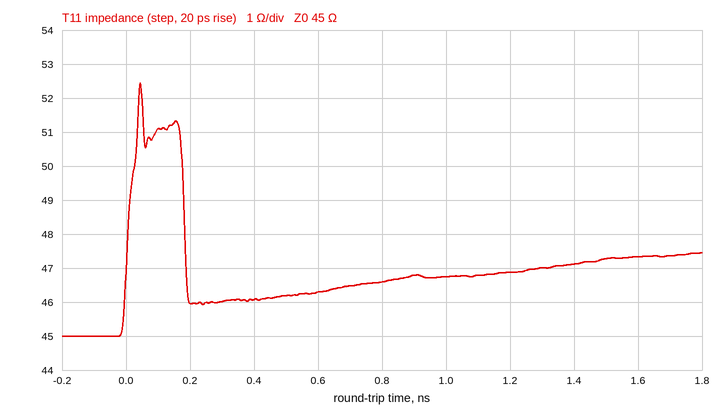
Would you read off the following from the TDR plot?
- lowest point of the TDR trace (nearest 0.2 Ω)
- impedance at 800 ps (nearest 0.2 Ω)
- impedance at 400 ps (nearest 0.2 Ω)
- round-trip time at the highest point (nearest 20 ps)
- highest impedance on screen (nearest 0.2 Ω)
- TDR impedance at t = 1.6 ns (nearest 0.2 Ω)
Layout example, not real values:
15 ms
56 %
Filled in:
45.0 Ω
46.6 Ω
46.0 Ω
40 ps
52.4 Ω
47.4 Ω
